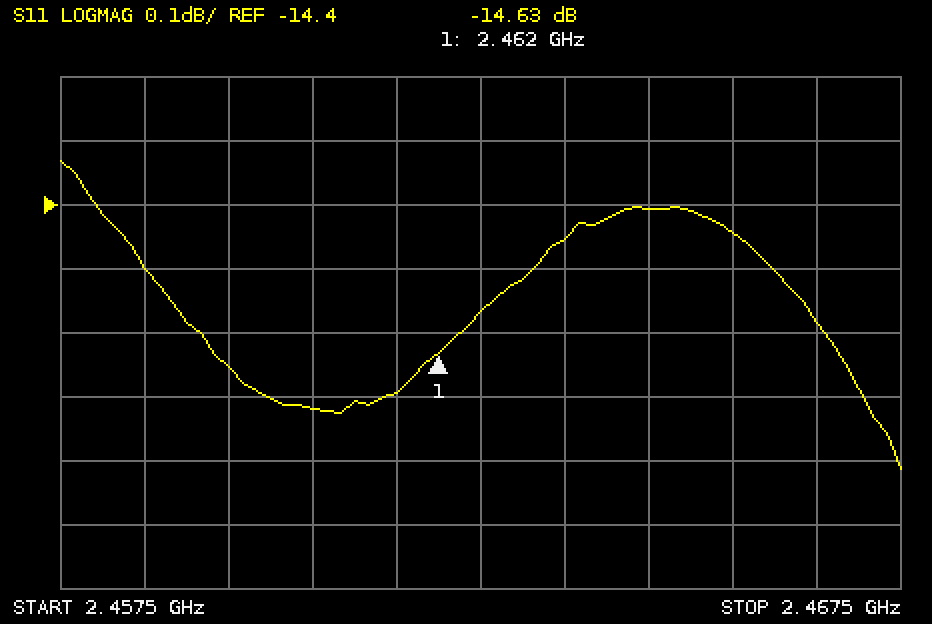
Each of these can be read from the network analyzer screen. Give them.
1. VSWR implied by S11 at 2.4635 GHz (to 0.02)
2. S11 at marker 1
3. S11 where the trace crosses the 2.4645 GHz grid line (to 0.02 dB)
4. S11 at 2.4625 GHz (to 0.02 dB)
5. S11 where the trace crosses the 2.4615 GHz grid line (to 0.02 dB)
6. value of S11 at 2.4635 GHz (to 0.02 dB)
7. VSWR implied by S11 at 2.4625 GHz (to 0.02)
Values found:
1.46
-14.63 dB
-14.40 dB
-14.56 dB
-14.70 dB
-14.46 dB
1.46
